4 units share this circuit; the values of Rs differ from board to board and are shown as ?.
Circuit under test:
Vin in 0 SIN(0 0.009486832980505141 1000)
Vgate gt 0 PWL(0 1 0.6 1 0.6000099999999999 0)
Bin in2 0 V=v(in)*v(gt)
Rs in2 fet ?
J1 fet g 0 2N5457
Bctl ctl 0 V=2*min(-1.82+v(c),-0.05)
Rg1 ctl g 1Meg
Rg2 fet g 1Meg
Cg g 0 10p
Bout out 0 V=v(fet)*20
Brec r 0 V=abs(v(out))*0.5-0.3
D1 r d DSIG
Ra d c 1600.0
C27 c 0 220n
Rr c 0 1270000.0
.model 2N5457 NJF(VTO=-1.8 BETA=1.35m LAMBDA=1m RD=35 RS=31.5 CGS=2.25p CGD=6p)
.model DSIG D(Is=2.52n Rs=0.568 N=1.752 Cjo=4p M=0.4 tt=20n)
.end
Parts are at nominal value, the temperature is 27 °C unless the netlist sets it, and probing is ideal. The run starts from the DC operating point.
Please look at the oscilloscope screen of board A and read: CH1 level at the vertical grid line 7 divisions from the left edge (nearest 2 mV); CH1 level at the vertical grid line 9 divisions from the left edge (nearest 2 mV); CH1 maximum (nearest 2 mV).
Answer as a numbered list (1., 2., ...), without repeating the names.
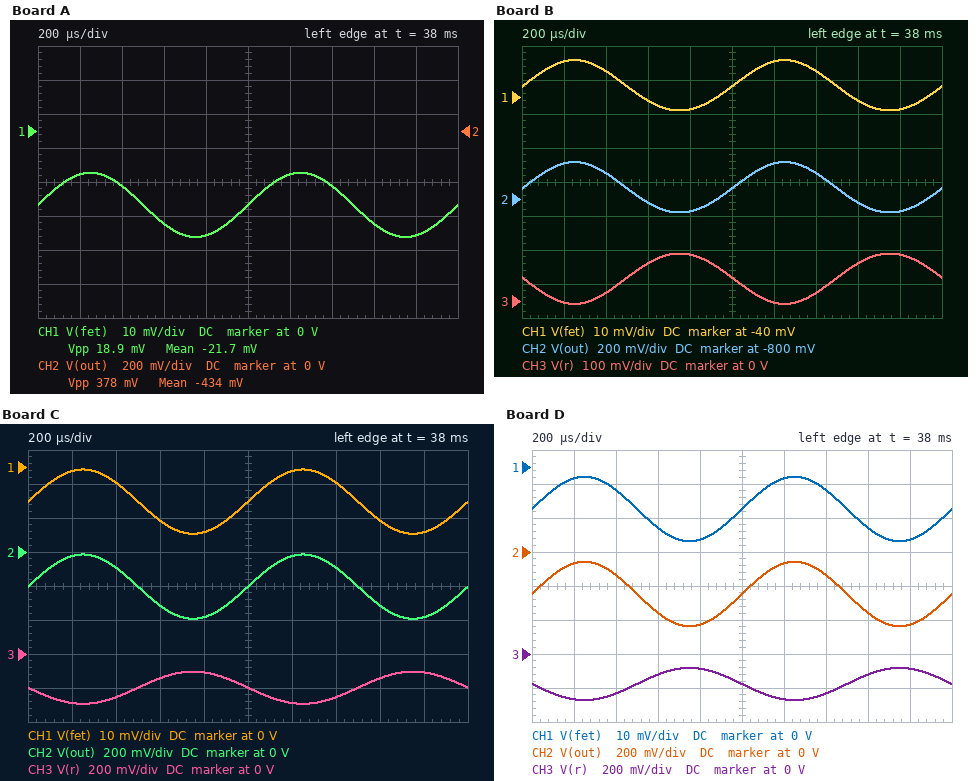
1. -16 mV
2. -30 mV
3. -12 mV
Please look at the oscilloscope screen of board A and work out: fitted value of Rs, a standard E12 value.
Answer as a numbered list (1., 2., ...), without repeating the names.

1. 12 kΩ
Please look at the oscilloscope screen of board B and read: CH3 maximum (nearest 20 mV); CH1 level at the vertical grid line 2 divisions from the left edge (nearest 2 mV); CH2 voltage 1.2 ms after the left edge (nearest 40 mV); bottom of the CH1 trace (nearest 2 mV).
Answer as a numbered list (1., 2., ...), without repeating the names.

1. 140 mV
2. -32 mV
3. -600 mV
4. -44 mV
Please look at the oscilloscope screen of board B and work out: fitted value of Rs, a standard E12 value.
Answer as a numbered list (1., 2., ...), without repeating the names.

1. 22 kΩ
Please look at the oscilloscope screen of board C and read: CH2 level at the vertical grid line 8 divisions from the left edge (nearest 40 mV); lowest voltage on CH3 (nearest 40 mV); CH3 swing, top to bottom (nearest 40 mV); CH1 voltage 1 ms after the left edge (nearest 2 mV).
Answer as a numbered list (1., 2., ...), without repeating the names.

1. -320 mV
2. -280 mV
3. 200 mV
4. -10 mV
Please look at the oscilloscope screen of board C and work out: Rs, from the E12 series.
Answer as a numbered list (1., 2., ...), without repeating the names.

1. 5.6 kΩ
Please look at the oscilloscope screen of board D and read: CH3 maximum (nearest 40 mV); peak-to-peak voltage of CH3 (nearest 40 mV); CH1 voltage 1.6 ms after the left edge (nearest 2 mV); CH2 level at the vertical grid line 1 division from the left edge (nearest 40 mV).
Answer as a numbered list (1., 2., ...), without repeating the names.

1. -80 mV
2. 200 mV
3. -18 mV
4. -80 mV
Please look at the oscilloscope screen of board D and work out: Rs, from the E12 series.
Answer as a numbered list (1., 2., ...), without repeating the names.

1. 6.8 kΩ
